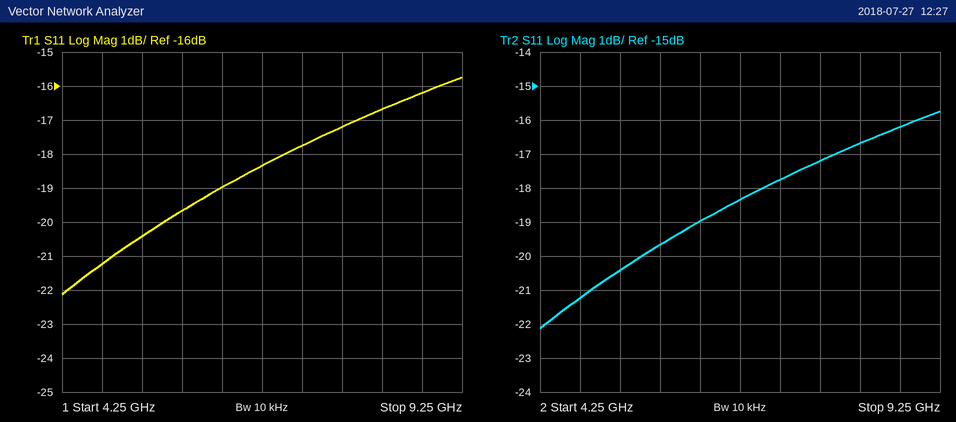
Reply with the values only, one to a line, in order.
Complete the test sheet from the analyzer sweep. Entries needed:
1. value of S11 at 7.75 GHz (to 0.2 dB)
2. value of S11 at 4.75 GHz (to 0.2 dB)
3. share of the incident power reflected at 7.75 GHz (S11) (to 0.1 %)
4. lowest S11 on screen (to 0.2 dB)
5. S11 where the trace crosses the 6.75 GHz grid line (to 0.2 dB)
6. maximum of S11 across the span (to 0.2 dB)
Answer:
-17.2 dB
-21.2 dB
1.9 %
-22.2 dB
-18.4 dB
-15.8 dB
